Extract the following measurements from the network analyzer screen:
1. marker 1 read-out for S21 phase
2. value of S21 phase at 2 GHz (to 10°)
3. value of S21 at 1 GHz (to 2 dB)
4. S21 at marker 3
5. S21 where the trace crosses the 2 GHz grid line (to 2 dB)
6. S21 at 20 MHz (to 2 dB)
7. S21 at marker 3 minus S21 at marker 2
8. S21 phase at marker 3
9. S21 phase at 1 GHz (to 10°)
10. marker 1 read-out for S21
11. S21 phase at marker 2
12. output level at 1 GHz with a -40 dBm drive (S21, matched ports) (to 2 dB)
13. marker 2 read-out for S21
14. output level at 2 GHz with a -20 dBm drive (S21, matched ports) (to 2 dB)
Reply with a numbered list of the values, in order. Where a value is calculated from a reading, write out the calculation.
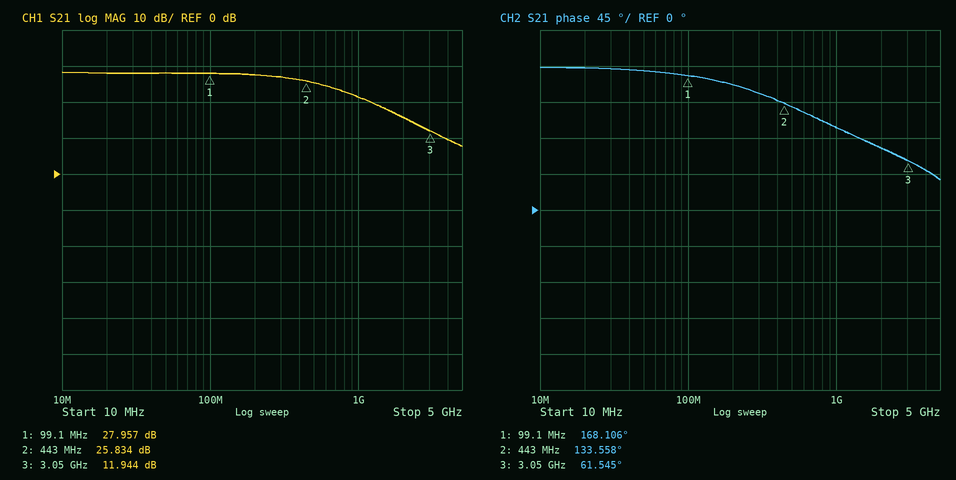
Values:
1. 168.106°
2. 80°
3. 22 dB
4. 11.944 dB
5. 16 dB
6. 28 dB
7. 11.944 − (25.834) = -13.890 dB
8. 61.545°
9. 100°
10. 27.957 dB
11. 133.558°
12. -40 dBm + (22 dB) = -18 dBm
13. 25.834 dB
14. -20 dBm + (16 dB) = -4 dBm
